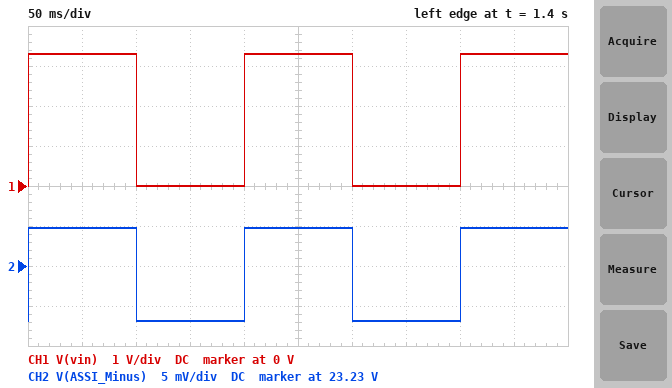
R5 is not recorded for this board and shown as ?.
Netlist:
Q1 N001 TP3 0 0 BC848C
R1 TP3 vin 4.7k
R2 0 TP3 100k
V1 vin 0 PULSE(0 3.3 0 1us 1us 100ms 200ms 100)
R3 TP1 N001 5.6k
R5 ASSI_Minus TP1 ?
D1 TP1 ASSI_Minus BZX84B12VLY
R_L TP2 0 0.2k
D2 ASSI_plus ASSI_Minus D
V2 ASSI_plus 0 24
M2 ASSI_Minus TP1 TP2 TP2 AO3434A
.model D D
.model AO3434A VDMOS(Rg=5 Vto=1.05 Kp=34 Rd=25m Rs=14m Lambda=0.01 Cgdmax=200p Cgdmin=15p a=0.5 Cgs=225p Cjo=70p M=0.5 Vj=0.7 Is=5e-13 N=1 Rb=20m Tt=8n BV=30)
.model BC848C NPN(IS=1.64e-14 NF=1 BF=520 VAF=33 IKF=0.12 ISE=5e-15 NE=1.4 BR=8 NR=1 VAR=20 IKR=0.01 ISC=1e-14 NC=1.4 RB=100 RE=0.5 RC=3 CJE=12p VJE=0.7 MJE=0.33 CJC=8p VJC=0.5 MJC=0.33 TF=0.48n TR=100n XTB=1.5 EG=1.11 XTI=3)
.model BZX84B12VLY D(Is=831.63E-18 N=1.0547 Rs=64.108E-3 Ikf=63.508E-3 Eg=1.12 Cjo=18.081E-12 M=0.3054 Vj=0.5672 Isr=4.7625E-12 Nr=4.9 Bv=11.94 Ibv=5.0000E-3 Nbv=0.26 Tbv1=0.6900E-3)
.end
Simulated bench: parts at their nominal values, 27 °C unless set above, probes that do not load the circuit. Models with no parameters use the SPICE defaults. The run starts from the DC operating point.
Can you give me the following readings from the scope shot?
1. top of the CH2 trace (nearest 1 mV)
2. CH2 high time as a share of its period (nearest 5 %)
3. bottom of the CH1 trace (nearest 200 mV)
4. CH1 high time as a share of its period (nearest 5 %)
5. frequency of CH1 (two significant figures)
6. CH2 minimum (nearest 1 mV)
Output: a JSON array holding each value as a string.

["23.235 V", "50 %", "0 V", "50 %", "5.0 Hz", "23.223 V"]
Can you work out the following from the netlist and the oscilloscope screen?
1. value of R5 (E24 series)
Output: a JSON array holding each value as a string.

["3.3 kΩ"]
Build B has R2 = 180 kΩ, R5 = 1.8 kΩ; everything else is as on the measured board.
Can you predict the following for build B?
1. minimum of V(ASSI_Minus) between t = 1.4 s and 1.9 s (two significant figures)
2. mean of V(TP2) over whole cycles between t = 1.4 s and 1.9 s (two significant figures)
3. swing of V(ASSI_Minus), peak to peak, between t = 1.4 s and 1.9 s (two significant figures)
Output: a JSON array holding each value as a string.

["23 V", "19 V", "6.6 mV"]
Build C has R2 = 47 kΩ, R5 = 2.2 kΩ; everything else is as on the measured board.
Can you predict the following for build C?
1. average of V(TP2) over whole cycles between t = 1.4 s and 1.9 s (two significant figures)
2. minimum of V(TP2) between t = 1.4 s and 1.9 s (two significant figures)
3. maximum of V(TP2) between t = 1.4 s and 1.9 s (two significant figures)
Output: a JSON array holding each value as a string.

["19 V", "16 V", "22 V"]
